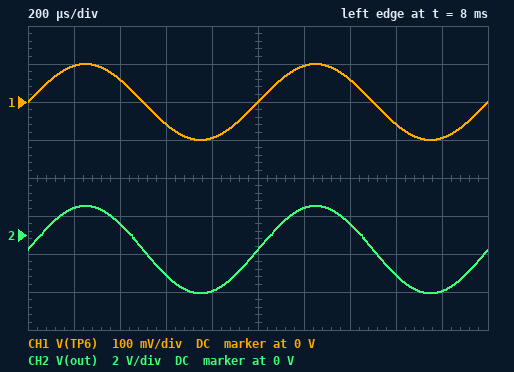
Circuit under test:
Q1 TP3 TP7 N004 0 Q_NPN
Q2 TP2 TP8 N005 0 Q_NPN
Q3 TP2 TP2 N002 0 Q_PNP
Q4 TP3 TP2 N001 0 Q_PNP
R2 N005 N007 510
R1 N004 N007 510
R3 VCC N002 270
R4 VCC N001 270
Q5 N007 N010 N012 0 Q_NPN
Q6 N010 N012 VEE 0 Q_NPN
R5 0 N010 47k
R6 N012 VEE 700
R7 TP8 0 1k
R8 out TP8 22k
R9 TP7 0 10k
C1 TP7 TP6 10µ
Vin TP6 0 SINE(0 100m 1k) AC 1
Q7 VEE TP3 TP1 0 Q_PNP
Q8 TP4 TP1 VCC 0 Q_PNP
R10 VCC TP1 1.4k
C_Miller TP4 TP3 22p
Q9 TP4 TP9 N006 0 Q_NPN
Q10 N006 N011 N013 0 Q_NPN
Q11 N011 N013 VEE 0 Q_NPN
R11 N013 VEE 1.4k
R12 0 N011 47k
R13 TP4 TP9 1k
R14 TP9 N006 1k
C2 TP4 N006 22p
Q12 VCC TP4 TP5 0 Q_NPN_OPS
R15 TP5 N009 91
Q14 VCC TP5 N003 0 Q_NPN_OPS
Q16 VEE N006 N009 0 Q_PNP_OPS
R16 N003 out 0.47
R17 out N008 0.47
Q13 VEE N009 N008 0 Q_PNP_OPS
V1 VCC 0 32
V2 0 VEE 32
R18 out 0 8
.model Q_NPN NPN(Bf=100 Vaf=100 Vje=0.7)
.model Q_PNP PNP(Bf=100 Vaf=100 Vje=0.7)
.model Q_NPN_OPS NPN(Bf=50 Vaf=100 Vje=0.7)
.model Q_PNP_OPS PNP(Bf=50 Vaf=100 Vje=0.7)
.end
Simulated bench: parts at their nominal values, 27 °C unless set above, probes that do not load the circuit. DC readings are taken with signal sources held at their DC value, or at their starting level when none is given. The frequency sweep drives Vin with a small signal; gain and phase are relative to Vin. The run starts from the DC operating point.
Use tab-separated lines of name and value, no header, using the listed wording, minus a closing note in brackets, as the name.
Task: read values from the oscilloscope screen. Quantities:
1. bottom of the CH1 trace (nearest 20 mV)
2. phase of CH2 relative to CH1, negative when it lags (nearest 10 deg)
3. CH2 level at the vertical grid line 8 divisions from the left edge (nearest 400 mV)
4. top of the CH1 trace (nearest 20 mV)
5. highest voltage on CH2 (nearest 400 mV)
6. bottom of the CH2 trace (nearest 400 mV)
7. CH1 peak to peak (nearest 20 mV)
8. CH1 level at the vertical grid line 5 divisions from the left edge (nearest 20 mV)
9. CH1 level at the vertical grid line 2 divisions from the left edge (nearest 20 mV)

bottom of the CH1 trace	-100 mV
phase of CH2 relative to CH1, negative when it lags	0 deg
CH2 level at the vertical grid line 8 divisions from the left edge	-2.0 V
top of the CH1 trace	100 mV
highest voltage on CH2	1.6 V
bottom of the CH2 trace	-3.2 V
CH1 peak to peak	200 mV
CH1 level at the vertical grid line 5 divisions from the left edge	0 V
CH1 level at the vertical grid line 2 divisions from the left edge	60 mV
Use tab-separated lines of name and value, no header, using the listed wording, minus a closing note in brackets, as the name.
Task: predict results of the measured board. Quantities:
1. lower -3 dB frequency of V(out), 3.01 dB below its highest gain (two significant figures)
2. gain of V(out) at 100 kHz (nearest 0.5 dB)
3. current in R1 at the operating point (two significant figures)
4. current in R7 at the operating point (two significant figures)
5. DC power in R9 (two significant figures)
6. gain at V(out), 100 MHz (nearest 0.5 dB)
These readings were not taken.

lower -3 dB frequency of V(out), 3.01 dB below its highest gain	1.6 Hz
gain of V(out) at 100 kHz	27.0 dB
current in R1 at the operating point	540 µA
current in R7 at the operating point	37 µA
DC power in R9	170 nW
gain at V(out), 100 MHz	-17.0 dB
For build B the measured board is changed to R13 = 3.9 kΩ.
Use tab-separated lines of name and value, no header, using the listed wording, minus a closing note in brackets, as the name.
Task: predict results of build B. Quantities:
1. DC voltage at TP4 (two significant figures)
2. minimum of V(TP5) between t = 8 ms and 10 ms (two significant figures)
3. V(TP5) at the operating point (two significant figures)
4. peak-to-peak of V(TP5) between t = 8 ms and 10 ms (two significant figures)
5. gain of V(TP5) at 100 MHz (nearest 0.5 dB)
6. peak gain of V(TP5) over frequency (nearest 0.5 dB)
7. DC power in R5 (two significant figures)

DC voltage at TP4	-370 mV
minimum of V(TP5) between t = 8 ms and 10 ms	-3.8 V
V(TP5) at the operating point	-1.2 V
peak-to-peak of V(TP5) between t = 8 ms and 10 ms	6.4 V
gain of V(TP5) at 100 MHz	-16.0 dB
peak gain of V(TP5) over frequency	28.5 dB
DC power in R5	20 mW
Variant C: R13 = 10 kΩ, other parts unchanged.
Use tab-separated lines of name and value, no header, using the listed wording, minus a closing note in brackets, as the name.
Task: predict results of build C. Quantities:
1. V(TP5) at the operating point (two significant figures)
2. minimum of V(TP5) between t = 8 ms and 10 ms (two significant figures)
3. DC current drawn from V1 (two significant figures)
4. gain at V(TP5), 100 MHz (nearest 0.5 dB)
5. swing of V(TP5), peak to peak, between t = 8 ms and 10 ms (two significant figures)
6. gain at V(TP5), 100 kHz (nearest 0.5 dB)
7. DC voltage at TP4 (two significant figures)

V(TP5) at the operating point	-260 mV
minimum of V(TP5) between t = 8 ms and 10 ms	-3.0 V
DC current drawn from V1	18 mA
gain at V(TP5), 100 MHz	-16.0 dB
swing of V(TP5), peak to peak, between t = 8 ms and 10 ms	5.5 V
gain at V(TP5), 100 kHz	28.5 dB
DC voltage at TP4	580 mV
